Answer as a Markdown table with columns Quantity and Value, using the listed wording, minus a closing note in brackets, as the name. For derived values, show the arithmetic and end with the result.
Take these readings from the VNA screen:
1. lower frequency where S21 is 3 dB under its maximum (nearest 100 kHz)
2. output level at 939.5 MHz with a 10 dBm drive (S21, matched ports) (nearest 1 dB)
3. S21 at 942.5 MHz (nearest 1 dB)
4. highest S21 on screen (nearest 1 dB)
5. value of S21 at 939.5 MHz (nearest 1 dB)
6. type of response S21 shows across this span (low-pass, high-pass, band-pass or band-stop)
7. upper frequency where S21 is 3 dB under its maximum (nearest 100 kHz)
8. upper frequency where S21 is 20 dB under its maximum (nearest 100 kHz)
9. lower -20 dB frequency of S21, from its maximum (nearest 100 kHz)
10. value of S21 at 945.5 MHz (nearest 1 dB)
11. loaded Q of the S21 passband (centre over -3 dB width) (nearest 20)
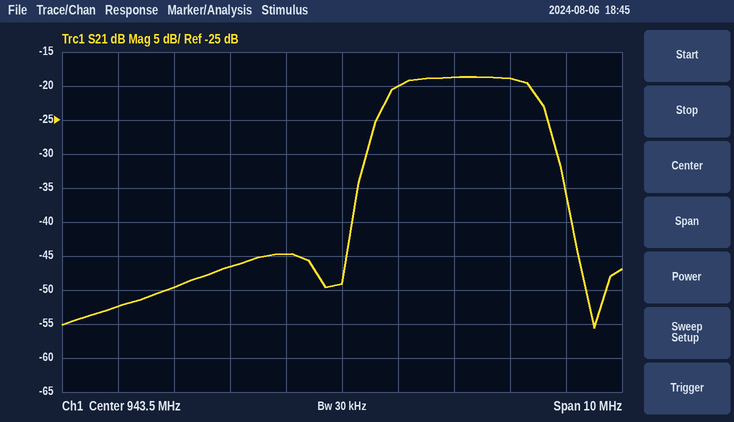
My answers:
| Quantity | Value |
|---|---|
| lower frequency where S21 is 3 dB under its maximum | 944.3 MHz |
| output level at 939.5 MHz with a 10 dBm drive (S21, matched ports) | 10 dBm + (-52 dB) = -42 dBm |
| S21 at 942.5 MHz | -45 dB |
| highest S21 on screen | -19 dB |
| value of S21 at 939.5 MHz | -52 dB |
| type of response S21 shows across this span | band-pass |
| upper frequency where S21 is 3 dB under its maximum | 947.0 MHz |
| upper frequency where S21 is 20 dB under its maximum | 947.6 MHz |
| lower -20 dB frequency of S21, from its maximum | 943.7 MHz |
| value of S21 at 945.5 MHz | -19 dB |
| loaded Q of the S21 passband (centre over -3 dB width) | 945.65 MHz / 2.7 MHz ≈ 350, so 360 to the nearest 20 |
